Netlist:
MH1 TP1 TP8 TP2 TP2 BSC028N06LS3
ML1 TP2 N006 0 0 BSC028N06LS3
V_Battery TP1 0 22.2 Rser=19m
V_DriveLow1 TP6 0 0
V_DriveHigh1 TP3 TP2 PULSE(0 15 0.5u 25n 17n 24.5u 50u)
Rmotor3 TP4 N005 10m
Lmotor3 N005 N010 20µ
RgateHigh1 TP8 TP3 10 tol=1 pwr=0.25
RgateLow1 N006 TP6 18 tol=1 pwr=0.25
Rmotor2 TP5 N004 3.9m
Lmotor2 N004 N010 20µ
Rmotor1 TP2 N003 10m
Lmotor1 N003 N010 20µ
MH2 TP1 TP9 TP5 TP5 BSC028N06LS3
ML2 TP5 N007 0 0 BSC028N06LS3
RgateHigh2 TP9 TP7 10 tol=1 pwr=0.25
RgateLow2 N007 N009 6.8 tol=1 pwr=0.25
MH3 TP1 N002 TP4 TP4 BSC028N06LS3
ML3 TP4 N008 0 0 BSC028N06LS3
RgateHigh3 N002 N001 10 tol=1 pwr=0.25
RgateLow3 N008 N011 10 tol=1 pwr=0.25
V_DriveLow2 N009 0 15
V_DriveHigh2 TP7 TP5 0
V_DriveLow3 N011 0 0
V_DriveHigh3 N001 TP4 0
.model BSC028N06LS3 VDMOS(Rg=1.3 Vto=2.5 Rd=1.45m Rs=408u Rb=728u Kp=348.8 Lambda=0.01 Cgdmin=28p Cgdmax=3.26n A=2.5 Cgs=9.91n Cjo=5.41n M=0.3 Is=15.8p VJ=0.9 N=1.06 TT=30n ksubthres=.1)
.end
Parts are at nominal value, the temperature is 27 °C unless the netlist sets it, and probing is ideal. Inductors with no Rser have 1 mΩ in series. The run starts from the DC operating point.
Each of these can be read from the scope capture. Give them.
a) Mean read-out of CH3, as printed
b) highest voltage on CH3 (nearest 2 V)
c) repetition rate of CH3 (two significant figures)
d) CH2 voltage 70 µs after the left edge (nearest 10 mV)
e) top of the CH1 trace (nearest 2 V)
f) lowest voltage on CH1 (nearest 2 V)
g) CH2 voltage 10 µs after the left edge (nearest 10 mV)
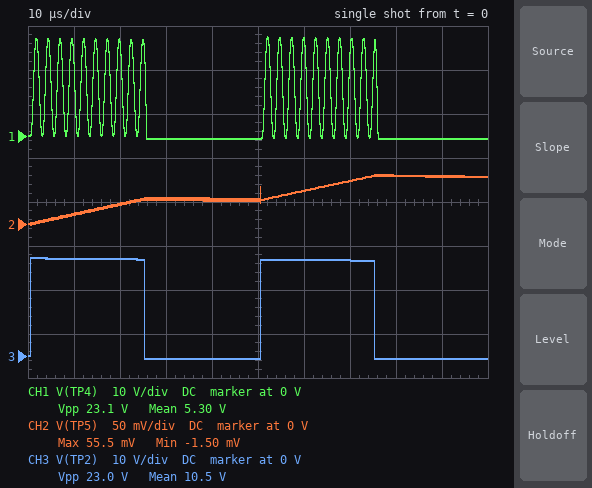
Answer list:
10.5 V
22 V
20 kHz
50 mV
22 V
0 V
10 mV
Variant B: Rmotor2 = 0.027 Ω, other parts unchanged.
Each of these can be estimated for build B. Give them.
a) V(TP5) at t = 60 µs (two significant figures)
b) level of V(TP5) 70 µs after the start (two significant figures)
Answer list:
37 mV
48 mV
